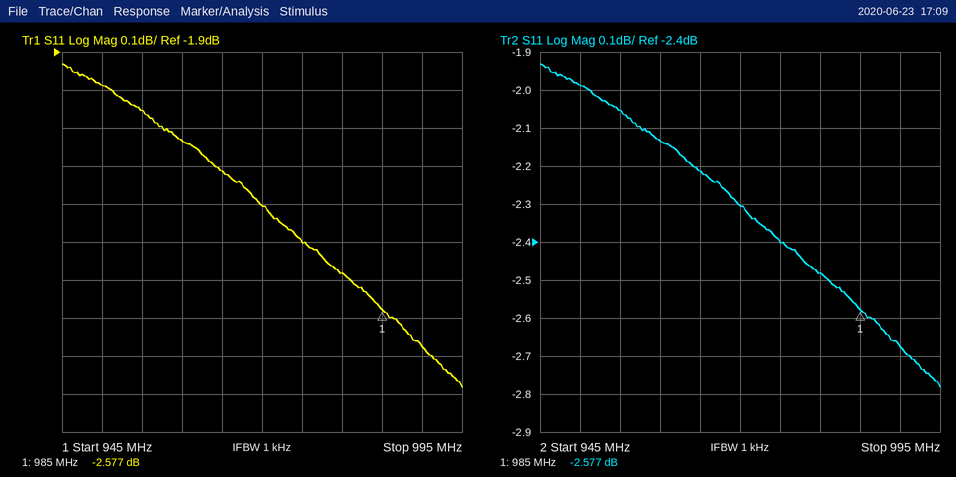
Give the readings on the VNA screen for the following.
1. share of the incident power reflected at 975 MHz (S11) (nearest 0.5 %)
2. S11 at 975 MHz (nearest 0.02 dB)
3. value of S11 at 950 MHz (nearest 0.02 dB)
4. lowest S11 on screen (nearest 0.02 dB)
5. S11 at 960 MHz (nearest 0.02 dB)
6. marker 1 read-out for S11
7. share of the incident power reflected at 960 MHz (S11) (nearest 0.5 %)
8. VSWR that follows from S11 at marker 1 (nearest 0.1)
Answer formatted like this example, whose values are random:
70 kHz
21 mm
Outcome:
57.5 %
-2.40 dB
-1.98 dB
-2.78 dB
-2.14 dB
-2.577 dB
61.0 %
6.8
